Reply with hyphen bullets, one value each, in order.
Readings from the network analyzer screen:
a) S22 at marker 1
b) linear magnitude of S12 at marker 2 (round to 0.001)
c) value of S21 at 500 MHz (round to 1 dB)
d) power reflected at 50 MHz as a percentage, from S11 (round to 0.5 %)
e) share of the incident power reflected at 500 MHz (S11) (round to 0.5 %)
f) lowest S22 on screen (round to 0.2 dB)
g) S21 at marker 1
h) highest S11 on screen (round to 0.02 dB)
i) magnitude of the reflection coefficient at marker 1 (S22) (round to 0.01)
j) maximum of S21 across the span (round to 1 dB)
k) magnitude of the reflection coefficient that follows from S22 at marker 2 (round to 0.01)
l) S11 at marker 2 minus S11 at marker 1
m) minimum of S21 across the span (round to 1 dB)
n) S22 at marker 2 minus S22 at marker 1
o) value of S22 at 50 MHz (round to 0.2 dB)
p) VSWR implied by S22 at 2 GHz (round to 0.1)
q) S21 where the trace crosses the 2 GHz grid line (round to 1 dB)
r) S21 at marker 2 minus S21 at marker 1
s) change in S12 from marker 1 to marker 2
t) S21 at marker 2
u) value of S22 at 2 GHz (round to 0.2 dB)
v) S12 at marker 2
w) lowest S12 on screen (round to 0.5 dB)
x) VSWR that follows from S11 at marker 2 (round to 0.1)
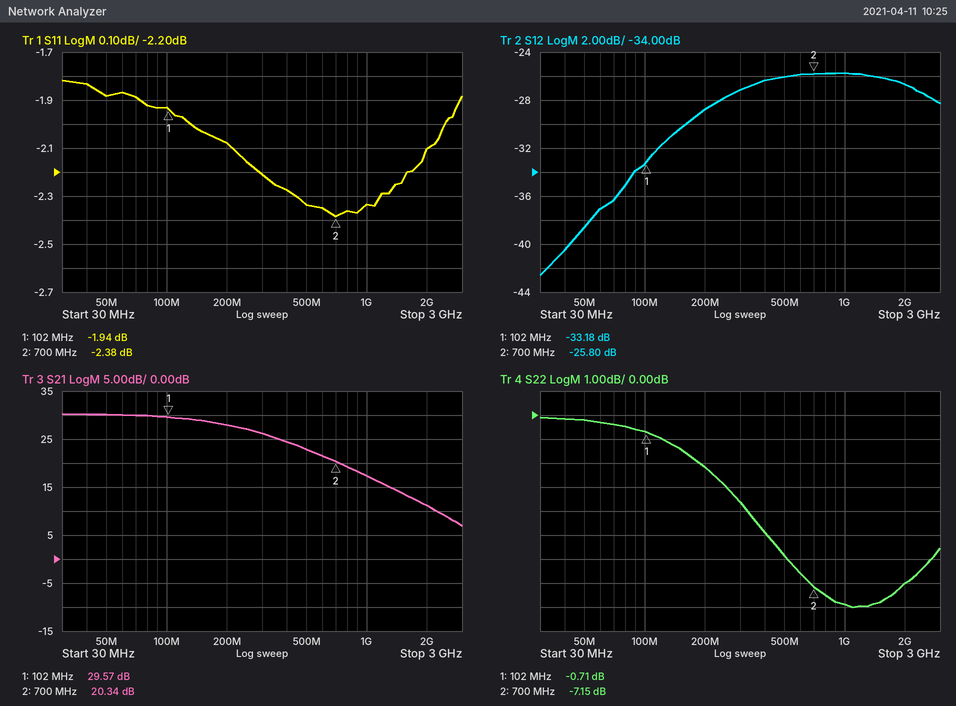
- -0.71 dB
- 0.051
- 23 dB
- 65.0 %
- 58.5 %
- -8.0 dB
- 29.57 dB
- -1.82 dB
- 0.92
- 30 dB
- 0.44
- -0.44 dB
- 7 dB
- -6.44 dB
- -0.2 dB
- 2.6
- 11 dB
- -9.23 dB
- 7.38 dB
- 20.34 dB
- -7.0 dB
- -25.80 dB
- -42.5 dB
- 7.3
